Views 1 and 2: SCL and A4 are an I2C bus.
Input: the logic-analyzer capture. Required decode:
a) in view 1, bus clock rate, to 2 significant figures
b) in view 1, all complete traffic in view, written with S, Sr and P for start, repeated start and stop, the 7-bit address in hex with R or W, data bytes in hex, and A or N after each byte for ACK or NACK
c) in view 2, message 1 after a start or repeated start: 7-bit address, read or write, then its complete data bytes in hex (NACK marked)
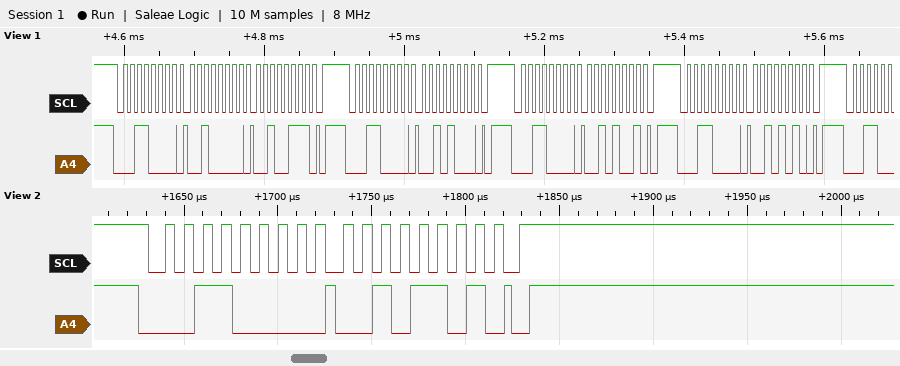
100 kHz
S 18W A 20 A 27 A P S 18W A 28 A P S 18W A 29 A P S 18W A 2A A P
0x18 write: 2D
